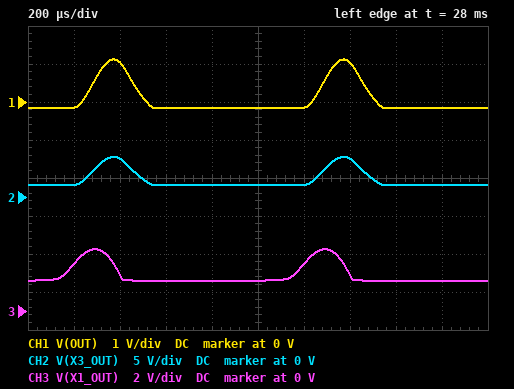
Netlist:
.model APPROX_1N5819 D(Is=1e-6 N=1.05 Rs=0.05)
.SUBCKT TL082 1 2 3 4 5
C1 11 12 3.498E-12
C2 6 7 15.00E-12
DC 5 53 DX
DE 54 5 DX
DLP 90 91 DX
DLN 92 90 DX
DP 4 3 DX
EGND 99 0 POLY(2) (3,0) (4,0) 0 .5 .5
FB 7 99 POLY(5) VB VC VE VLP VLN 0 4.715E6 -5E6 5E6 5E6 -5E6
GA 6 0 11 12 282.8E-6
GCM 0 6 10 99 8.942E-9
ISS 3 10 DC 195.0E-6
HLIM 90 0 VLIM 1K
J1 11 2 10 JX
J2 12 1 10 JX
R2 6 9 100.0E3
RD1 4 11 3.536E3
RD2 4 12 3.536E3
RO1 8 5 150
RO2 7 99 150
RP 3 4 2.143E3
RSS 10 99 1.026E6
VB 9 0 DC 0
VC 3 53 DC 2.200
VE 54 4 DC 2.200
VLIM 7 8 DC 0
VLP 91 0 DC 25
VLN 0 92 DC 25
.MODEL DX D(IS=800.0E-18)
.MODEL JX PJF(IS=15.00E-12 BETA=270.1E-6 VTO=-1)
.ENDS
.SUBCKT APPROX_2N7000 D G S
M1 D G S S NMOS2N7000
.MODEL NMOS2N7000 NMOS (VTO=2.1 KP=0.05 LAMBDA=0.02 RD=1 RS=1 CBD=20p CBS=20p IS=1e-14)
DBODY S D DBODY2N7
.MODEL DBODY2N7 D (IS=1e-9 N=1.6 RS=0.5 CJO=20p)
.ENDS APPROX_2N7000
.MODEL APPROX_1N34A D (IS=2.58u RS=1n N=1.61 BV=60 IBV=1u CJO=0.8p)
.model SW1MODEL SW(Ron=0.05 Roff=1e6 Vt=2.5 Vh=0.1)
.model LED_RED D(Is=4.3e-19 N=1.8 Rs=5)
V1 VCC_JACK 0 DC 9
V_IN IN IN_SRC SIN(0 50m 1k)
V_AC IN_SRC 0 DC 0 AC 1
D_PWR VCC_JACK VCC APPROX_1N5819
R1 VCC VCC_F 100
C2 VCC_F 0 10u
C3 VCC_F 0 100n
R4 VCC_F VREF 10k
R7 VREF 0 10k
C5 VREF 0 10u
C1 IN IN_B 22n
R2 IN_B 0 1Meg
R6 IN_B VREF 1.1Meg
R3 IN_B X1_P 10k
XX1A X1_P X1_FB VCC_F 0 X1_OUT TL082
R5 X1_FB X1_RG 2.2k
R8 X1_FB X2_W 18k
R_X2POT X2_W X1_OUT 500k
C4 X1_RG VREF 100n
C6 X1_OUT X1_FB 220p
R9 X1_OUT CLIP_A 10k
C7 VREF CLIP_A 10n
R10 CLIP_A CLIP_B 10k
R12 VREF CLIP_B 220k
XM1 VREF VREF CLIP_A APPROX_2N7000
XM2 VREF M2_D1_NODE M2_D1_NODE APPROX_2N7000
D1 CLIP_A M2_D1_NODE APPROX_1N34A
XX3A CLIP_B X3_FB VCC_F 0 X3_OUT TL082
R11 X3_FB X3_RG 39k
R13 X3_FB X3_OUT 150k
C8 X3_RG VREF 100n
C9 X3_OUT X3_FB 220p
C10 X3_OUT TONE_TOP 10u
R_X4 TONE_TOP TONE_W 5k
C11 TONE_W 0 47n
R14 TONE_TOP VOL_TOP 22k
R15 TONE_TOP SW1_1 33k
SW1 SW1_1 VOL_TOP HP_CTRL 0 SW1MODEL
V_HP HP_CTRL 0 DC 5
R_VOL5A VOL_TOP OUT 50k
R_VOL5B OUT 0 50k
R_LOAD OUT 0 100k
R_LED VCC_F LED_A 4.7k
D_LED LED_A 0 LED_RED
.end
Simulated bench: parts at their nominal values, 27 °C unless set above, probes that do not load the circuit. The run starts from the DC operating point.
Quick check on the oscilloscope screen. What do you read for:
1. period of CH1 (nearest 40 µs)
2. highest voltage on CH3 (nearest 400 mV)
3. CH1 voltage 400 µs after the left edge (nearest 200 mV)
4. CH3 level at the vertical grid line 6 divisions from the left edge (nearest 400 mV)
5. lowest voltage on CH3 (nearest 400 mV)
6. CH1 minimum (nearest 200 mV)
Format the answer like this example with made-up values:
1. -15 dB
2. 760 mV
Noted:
1. 1.00 ms
2. 3.2 V
3. 1.0 V
4. 2.4 V
5. 1.6 V
6. -200 mV
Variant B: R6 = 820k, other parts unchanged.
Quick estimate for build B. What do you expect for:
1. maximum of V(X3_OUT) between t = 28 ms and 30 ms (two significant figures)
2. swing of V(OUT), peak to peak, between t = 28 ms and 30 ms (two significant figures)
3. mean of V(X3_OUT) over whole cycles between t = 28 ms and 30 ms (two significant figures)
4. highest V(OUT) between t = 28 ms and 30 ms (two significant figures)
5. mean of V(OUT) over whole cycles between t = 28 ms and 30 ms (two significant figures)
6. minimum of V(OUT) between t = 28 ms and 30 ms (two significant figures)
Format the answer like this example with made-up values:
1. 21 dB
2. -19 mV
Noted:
1. 6.3 V
2. 1.6 V
3. 2.6 V
4. 1.4 V
5. 110 mV
6. -260 mV
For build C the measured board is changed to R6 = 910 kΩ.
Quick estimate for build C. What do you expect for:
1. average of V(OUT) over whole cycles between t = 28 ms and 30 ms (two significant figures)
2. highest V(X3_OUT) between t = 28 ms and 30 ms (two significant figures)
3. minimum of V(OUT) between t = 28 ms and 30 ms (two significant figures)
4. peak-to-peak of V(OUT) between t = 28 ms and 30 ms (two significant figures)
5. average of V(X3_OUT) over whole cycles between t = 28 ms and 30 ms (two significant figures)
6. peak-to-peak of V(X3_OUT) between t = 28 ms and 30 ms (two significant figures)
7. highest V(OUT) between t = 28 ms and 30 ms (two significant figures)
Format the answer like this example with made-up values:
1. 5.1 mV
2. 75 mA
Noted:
1. 110 mV
2. 6.3 V
3. -230 mV
4. 1.6 V
5. 2.5 V
6. 4.7 V
7. 1.4 V
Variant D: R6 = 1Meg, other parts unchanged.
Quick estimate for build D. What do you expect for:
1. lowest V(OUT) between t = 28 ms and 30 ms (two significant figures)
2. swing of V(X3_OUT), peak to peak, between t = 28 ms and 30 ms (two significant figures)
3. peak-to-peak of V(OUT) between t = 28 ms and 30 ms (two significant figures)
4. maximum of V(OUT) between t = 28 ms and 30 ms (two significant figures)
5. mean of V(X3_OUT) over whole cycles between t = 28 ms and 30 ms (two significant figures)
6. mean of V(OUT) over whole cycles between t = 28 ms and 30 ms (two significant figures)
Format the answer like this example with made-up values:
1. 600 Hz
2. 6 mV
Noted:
1. -200 mV
2. 4.5 V
3. 1.6 V
4. 1.4 V
5. 2.4 V
6. 91 mV
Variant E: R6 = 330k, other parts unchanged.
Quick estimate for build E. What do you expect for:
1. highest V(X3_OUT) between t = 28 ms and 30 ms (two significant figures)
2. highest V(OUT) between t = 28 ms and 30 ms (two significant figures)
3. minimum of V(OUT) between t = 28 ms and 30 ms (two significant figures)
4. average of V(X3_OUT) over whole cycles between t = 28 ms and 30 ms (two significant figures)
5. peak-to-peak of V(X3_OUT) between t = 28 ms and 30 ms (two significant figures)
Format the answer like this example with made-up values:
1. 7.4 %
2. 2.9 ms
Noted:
1. 6.3 V
2. 1.1 V
3. -510 mV
4. 3.1 V
5. 4.8 V
